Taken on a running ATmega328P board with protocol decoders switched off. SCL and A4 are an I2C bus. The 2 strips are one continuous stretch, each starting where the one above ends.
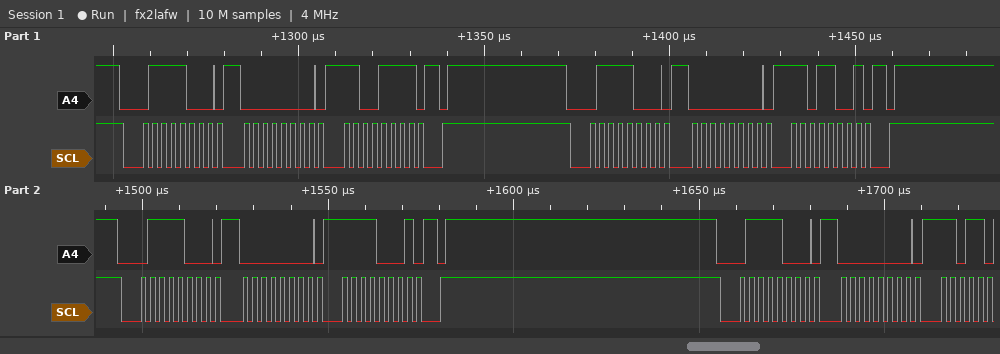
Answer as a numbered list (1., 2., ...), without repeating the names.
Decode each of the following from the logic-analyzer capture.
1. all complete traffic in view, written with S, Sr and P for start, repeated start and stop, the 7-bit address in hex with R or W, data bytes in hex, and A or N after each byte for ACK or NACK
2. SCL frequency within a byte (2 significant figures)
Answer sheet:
1. S 3CW A 00 A CF A P S 3CW A 00 A D9 A P S 3CW A 00 A F1 A P S 3CW A 00 A
2. 400 kHz
